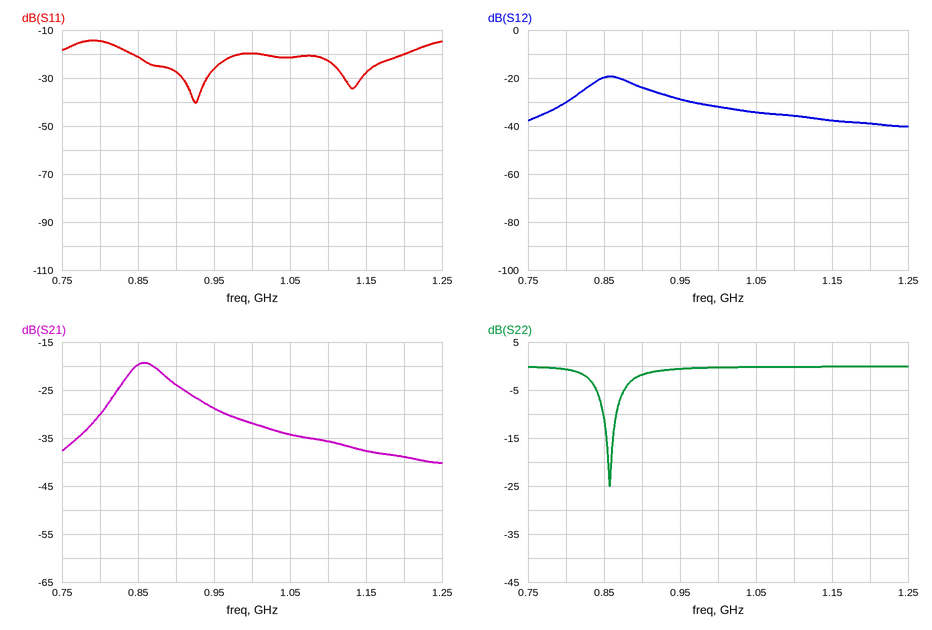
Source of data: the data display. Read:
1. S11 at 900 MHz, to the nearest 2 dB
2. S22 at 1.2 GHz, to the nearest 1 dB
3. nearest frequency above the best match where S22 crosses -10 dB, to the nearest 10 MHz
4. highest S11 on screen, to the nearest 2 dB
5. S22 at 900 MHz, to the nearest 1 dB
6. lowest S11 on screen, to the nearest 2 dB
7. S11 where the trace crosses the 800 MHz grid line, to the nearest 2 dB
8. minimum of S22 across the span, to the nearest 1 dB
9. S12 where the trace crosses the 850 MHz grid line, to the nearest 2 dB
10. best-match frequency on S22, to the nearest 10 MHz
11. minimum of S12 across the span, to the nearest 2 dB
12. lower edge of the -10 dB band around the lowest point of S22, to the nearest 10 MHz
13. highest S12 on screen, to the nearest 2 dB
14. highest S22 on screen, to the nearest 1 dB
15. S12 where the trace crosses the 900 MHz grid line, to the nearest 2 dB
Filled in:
-28 dB
0 dB
870 MHz
-14 dB
-2 dB
-40 dB
-14 dB
-25 dB
-20 dB
860 MHz
-40 dB
850 MHz
-20 dB
0 dB
-24 dB
